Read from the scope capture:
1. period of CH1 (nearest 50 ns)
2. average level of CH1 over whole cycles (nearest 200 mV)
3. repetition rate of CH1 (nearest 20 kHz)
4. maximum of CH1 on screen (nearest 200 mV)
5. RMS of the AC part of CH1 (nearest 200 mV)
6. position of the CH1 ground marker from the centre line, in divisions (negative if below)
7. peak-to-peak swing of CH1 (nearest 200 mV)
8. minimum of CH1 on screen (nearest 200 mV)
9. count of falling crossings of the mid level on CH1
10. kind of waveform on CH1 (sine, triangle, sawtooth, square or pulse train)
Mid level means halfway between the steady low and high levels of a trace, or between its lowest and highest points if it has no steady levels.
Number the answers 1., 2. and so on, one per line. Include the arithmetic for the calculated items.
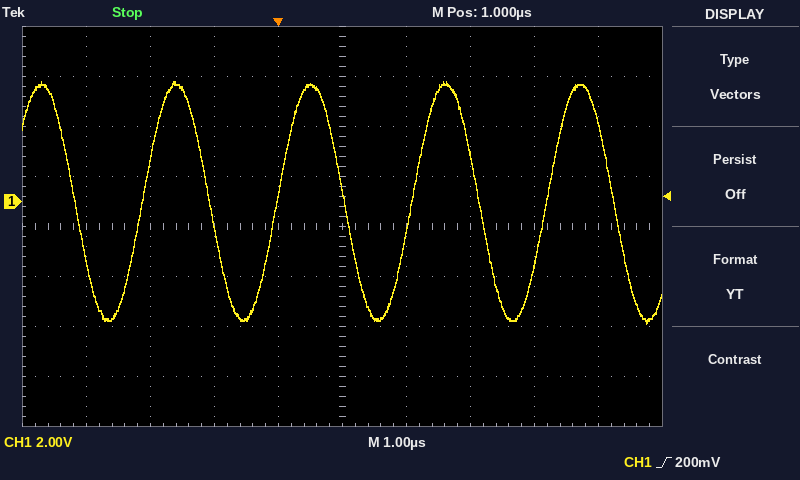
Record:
1. 2.10 µs
2. (4.8 V + (-4.8 V)) / 2 ≈ 0.0 V
3. 1 / 2.10 µs ≈ 476 kHz, so 480 kHz to the nearest 20 kHz
4. 4.8 V
5. 9.6 V / (2√2) ≈ 3.4 V
6. +0.5 div
7. 4.8 V − (-4.8 V) = 9.6 V
8. -4.8 V
9. 5
10. sine
